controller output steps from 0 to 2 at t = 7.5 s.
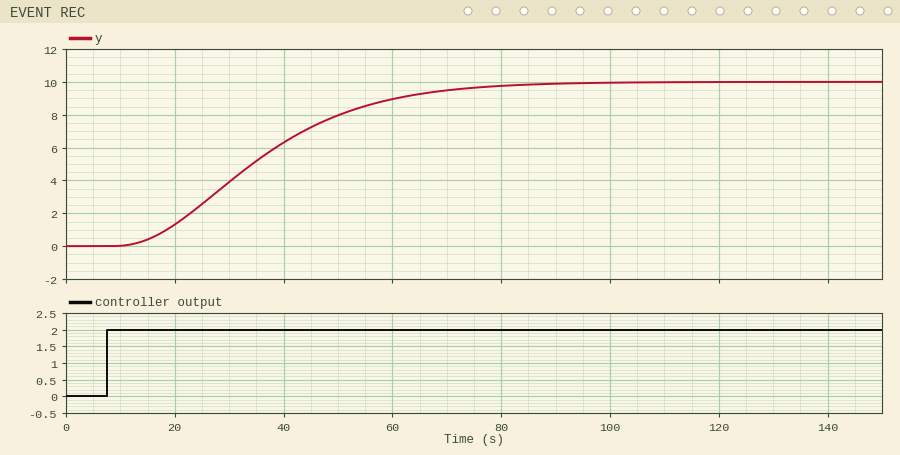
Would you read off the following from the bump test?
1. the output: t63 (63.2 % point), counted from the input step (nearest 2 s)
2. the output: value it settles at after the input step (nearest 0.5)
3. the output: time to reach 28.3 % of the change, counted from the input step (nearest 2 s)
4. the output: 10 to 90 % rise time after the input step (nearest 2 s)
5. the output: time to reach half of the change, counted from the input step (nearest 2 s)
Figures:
32 s
10.0
18 s
42 s
26 s
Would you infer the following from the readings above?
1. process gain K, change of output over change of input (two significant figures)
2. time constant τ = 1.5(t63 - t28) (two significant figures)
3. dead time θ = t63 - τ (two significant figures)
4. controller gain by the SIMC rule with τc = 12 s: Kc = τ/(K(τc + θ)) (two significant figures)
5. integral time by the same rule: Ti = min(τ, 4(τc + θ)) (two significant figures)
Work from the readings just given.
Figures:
5.0
21 s
11 s
0.18
21 s
